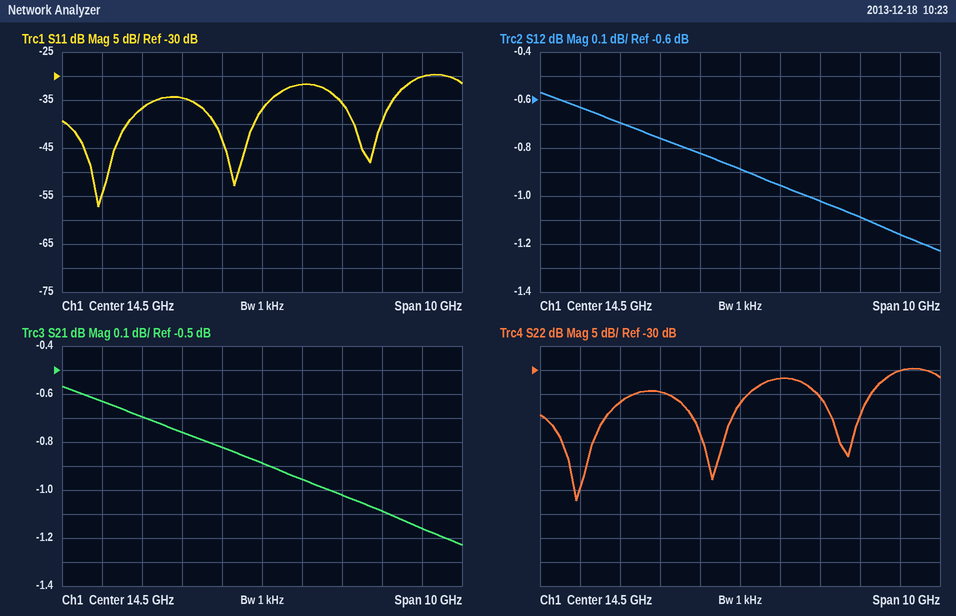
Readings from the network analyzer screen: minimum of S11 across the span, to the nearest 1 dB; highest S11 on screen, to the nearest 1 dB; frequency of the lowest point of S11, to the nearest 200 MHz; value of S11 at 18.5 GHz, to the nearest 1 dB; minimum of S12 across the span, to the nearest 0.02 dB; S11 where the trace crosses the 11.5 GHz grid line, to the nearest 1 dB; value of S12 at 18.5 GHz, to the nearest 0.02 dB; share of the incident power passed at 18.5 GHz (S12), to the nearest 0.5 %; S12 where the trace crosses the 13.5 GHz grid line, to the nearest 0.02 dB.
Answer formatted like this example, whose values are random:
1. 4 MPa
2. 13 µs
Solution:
1. -57 dB
2. -30 dB
3. 10.4 GHz
4. -30 dB
5. -1.22 dB
6. -37 dB
7. -1.16 dB
8. 76.5 %
9. -0.82 dB
